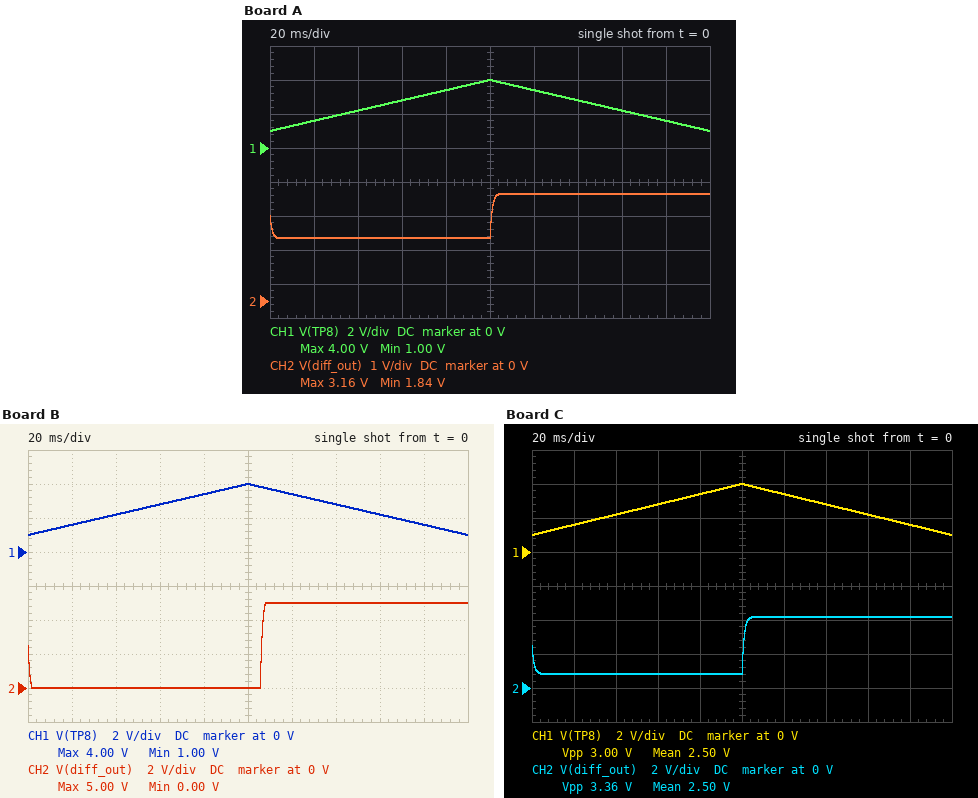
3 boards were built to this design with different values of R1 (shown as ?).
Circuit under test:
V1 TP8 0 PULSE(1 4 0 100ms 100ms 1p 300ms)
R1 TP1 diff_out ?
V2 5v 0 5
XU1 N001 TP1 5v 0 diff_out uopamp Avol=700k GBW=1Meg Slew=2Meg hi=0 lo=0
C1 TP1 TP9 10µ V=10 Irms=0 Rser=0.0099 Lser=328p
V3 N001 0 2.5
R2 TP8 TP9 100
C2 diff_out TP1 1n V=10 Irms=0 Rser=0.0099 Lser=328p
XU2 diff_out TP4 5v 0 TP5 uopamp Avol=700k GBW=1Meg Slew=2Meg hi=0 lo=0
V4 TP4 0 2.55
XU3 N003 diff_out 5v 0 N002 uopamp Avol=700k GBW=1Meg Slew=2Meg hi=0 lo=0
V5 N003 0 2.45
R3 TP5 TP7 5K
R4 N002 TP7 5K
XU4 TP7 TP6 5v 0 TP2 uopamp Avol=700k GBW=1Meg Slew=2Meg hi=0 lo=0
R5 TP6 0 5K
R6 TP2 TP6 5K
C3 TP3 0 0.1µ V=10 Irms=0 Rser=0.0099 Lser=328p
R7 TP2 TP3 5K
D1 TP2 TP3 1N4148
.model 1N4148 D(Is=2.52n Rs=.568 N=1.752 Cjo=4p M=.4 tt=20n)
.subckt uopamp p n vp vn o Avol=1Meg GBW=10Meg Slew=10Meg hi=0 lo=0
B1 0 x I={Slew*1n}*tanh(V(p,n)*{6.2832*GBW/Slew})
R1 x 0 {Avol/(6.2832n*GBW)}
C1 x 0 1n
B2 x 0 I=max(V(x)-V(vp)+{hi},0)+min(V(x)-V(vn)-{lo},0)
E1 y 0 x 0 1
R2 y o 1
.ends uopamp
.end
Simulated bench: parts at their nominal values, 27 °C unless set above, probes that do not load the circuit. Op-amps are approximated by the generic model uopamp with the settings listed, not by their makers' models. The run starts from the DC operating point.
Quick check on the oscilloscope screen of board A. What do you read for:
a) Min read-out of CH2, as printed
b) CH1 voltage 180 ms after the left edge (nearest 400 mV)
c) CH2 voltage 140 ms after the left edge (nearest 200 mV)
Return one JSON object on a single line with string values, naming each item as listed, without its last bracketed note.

{"Min read-out of CH2, as printed": "1.84 V", "CH1 voltage 180 ms after the left edge": "1.6 V", "CH2 voltage 140 ms after the left edge": "3.2 V"}
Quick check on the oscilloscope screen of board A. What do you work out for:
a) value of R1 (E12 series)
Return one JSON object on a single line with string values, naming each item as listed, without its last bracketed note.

{"value of R1": "2.2 kΩ"}
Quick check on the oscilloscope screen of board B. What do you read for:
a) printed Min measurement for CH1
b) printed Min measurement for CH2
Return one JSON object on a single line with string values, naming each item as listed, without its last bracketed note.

{"printed Min measurement for CH1": "1.00 V", "printed Min measurement for CH2": "0.00 V"}
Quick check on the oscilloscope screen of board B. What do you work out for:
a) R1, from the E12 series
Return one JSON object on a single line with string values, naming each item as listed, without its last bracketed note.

{"R1, from the E12 series": "10 kΩ"}
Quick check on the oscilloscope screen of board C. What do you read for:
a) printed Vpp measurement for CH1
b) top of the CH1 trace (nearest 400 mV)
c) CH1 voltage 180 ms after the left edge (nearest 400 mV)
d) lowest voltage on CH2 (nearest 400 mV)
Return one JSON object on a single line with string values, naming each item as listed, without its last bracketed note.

{"printed Vpp measurement for CH1": "3.00 V", "top of the CH1 trace": "4.0 V", "CH1 voltage 180 ms after the left edge": "1.6 V", "lowest voltage on CH2": "800 mV"}
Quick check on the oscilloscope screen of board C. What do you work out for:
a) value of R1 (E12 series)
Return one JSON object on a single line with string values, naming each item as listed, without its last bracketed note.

{"value of R1": "5.6 kΩ"}
